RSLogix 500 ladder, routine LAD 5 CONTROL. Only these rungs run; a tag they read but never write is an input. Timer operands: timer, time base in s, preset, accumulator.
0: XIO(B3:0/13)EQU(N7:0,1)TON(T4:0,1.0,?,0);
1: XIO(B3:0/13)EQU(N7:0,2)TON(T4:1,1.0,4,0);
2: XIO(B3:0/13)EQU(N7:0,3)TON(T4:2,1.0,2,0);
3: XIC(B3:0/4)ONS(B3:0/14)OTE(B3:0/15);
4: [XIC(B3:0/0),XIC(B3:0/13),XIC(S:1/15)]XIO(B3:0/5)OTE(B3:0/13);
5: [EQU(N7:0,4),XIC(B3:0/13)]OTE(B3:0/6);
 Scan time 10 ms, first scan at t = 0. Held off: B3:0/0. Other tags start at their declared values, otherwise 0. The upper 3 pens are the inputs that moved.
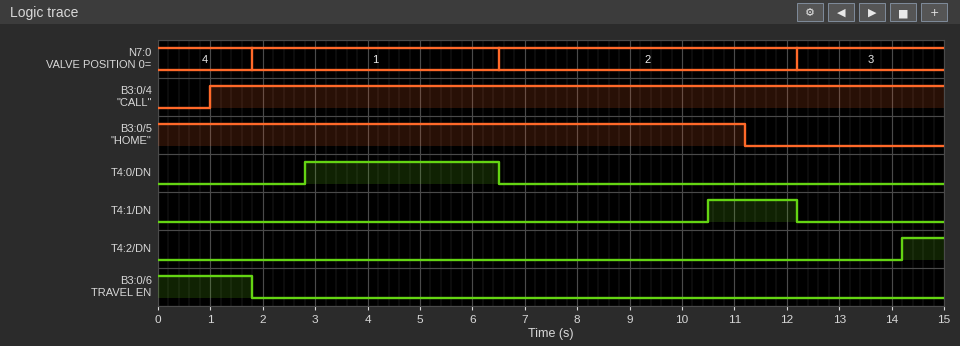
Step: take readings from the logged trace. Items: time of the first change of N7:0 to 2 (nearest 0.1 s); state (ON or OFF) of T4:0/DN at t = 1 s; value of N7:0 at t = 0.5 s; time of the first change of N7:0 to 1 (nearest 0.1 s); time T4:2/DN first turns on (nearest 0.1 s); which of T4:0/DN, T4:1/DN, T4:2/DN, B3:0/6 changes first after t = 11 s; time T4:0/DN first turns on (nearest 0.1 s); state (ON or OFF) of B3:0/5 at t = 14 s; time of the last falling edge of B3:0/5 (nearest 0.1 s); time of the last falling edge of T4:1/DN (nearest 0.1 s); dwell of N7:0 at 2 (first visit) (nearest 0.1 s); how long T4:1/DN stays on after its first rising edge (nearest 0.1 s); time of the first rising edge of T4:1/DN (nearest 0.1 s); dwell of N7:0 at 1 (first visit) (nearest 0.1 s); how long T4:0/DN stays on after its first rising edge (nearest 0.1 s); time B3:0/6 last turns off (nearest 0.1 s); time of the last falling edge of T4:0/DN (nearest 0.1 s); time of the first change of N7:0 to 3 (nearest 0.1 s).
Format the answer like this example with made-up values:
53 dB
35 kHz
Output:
6.5 s
OFF
4
1.8 s
14.2 s
T4:1/DN
2.8 s
OFF
11.2 s
12.2 s
5.7 s
1.7 s
10.5 s
4.7 s
3.7 s
1.8 s
6.5 s
12.2 s
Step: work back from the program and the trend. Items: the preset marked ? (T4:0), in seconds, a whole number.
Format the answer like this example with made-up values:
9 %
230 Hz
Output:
1 s
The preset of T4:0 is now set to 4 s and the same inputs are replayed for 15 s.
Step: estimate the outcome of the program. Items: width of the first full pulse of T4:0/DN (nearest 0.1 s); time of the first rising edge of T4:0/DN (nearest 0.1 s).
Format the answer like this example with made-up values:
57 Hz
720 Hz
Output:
0.7 s
5.8 s
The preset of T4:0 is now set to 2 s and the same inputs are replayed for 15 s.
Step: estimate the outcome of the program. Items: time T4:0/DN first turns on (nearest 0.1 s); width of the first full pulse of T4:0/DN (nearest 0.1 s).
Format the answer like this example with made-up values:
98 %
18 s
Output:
3.8 s
2.7 s
